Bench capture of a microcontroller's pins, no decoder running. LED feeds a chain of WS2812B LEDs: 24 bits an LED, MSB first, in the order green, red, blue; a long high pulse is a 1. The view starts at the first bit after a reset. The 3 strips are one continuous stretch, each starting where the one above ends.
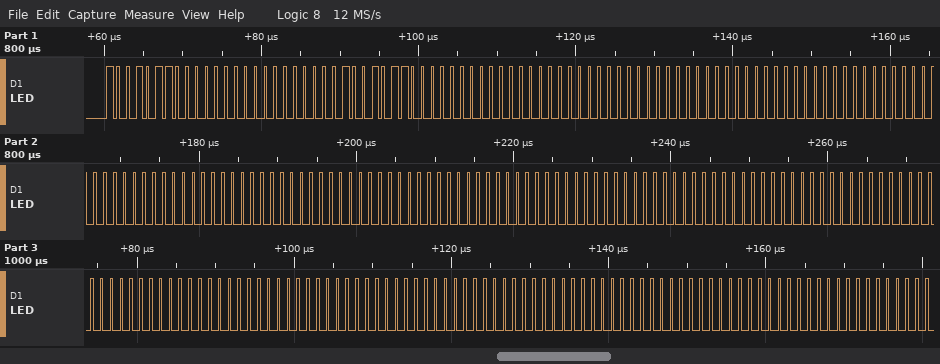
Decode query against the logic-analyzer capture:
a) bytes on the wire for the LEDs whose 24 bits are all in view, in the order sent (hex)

96 00 00 96 00 00 00 00 00 00 00 00 00 00 00 00 00 00 00 00 00 00 00 00 00 00 00 00 00 00
